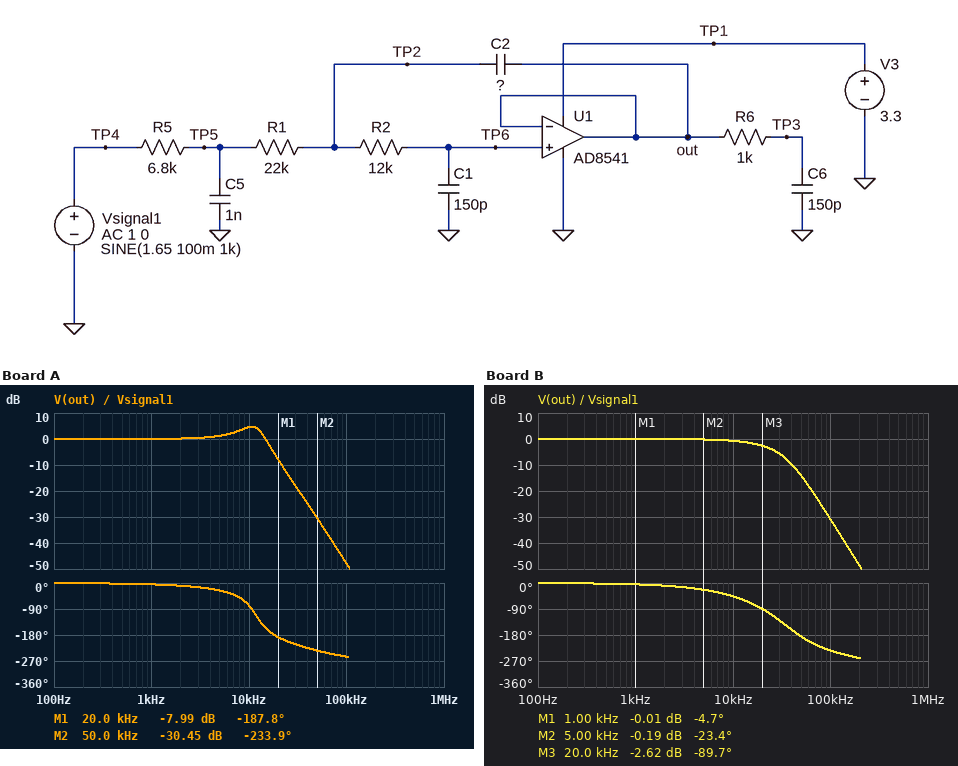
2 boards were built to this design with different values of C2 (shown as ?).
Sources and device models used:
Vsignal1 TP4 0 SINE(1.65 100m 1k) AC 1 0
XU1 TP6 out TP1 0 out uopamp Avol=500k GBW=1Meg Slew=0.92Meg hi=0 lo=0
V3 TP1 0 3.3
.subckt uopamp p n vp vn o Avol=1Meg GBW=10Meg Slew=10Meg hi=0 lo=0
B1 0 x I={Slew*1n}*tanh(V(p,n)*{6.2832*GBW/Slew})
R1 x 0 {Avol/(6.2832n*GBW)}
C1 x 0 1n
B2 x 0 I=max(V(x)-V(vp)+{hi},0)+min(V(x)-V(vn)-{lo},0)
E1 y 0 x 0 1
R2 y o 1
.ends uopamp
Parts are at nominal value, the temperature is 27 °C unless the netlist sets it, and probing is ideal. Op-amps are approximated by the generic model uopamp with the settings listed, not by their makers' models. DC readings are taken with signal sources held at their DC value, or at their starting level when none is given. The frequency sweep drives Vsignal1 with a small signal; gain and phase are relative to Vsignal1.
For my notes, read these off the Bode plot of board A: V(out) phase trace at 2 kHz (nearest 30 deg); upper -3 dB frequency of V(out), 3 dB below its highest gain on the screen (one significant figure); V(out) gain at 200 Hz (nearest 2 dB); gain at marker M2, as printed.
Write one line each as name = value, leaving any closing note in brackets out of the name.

V(out) phase trace at 2 kHz = 0 deg
upper -3 dB frequency of V(out), 3 dB below its highest gain on the screen = 10 kHz
V(out) gain at 200 Hz = 0 dB
gain at marker M2, as printed = -30.45 dB
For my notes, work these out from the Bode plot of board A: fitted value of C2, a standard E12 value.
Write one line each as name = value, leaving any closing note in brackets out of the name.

fitted value of C2, a standard E12 value = 3.3 nF
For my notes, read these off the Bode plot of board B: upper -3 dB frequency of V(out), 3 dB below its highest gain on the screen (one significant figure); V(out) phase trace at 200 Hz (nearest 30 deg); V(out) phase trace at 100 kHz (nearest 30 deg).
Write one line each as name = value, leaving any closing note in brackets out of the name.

upper -3 dB frequency of V(out), 3 dB below its highest gain on the screen = 20 kHz
V(out) phase trace at 200 Hz = 0 deg
V(out) phase trace at 100 kHz = -240 deg
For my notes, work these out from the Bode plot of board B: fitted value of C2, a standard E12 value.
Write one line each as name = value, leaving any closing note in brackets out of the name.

fitted value of C2, a standard E12 value = 470 pF
